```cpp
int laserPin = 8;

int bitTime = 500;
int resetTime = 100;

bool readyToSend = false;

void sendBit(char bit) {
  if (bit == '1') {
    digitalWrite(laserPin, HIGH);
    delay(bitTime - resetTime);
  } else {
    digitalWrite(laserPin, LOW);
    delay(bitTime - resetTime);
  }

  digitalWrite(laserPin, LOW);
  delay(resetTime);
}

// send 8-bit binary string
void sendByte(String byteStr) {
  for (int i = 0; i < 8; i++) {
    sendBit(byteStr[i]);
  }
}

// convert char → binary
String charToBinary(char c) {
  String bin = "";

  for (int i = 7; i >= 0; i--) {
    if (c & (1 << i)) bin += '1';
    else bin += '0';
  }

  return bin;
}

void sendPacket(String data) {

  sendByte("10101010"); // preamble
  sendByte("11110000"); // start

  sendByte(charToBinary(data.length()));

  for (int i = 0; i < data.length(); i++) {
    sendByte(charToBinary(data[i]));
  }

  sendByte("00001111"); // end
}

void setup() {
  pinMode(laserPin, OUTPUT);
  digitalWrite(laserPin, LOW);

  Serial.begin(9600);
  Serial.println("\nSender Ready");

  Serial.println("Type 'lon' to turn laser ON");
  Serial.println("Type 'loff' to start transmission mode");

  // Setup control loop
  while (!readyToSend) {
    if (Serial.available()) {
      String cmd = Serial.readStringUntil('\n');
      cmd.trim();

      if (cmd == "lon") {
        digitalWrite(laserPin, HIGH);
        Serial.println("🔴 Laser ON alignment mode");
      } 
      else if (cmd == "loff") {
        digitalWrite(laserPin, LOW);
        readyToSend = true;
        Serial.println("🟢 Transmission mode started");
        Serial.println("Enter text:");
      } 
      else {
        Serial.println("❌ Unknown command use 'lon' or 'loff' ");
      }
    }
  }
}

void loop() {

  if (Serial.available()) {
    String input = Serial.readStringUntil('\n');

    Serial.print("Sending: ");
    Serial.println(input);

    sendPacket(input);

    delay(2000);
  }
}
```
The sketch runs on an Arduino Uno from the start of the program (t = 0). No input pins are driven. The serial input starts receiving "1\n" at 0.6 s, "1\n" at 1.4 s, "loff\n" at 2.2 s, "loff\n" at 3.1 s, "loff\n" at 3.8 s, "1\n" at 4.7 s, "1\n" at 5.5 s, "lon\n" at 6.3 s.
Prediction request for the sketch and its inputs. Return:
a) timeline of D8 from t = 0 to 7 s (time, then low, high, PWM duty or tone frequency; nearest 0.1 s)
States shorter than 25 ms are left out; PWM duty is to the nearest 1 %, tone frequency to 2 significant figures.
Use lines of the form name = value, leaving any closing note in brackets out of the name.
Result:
timeline of D8 from t = 0 to 7 s = 0 s low; 3.1 s high; 3.5 s low; 4.1 s high; 4.5 s low; 5.1 s high; 5.5 s low; 6.1 s high; 6.5 s low
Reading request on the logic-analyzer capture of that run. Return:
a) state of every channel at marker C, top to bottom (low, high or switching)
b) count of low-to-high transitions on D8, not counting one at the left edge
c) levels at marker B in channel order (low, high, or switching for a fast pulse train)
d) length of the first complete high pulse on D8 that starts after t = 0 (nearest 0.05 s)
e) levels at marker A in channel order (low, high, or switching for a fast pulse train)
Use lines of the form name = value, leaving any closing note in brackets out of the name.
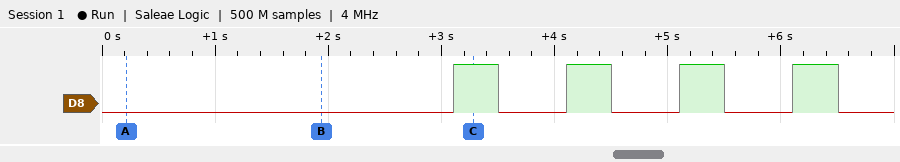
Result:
state of every channel at marker C, top to bottom = D8 high
count of low-to-high transitions on D8, not counting one at the left edge = 4
levels at marker B in channel order = D8 low
length of the first complete high pulse on D8 that starts after t = 0 = 0.40 s
levels at marker A in channel order = D8 low
